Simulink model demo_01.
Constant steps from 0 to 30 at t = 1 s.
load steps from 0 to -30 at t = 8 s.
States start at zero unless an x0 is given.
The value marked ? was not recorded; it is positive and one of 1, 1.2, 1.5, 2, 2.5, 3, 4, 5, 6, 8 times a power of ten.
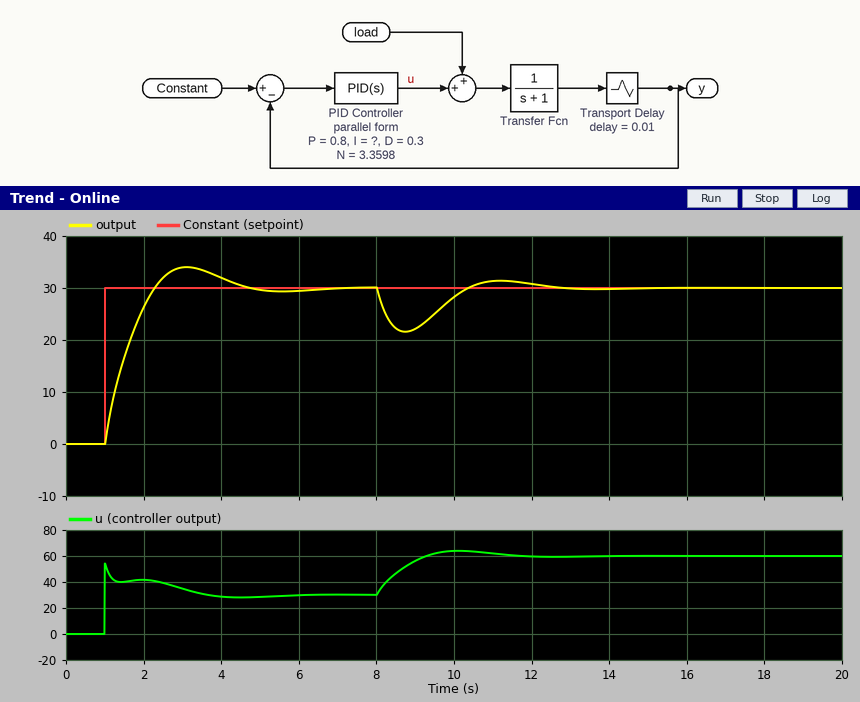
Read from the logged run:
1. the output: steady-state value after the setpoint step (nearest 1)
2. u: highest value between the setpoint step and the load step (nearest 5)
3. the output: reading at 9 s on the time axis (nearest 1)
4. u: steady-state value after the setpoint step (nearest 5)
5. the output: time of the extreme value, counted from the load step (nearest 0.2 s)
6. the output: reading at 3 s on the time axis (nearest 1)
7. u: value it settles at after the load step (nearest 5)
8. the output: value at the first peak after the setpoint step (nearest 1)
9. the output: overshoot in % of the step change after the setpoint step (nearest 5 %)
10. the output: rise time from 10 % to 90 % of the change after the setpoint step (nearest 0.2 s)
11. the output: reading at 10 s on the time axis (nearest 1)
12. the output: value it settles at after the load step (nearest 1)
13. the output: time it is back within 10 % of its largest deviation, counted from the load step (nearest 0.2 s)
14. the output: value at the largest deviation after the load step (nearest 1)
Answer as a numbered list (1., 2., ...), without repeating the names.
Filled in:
1. 30
2. 55
3. 22
4. 30
5. 0.8 s
6. 34
7. 60
8. 34
9. 15 %
10. 1.0 s
11. 28
12. 30
13. 4.0 s
14. 22
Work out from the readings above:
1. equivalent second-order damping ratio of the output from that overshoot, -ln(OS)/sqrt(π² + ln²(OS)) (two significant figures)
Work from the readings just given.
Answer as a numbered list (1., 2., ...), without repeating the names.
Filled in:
1. 0.52
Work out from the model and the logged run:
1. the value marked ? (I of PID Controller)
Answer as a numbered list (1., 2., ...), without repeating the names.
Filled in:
1. 3
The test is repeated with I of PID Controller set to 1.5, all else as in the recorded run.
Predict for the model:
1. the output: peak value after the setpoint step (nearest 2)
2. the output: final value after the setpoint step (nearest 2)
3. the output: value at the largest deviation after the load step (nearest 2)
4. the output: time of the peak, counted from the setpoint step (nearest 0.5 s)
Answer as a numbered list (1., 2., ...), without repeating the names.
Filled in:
1. 32
2. 30
3. 20
4. 3.5 s
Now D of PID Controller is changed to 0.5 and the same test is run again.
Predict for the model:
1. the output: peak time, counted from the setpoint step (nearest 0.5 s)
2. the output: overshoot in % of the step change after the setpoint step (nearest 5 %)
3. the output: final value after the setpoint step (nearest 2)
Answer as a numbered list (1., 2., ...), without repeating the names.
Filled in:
1. 2.5 s
2. 10 %
3. 30
